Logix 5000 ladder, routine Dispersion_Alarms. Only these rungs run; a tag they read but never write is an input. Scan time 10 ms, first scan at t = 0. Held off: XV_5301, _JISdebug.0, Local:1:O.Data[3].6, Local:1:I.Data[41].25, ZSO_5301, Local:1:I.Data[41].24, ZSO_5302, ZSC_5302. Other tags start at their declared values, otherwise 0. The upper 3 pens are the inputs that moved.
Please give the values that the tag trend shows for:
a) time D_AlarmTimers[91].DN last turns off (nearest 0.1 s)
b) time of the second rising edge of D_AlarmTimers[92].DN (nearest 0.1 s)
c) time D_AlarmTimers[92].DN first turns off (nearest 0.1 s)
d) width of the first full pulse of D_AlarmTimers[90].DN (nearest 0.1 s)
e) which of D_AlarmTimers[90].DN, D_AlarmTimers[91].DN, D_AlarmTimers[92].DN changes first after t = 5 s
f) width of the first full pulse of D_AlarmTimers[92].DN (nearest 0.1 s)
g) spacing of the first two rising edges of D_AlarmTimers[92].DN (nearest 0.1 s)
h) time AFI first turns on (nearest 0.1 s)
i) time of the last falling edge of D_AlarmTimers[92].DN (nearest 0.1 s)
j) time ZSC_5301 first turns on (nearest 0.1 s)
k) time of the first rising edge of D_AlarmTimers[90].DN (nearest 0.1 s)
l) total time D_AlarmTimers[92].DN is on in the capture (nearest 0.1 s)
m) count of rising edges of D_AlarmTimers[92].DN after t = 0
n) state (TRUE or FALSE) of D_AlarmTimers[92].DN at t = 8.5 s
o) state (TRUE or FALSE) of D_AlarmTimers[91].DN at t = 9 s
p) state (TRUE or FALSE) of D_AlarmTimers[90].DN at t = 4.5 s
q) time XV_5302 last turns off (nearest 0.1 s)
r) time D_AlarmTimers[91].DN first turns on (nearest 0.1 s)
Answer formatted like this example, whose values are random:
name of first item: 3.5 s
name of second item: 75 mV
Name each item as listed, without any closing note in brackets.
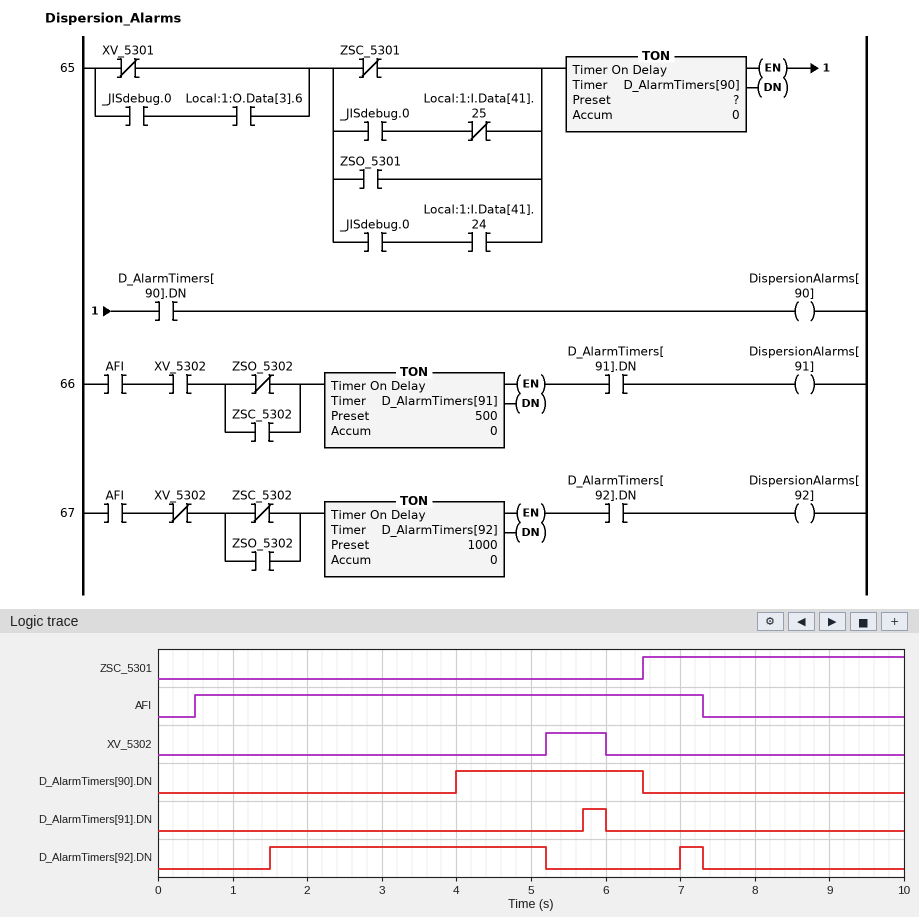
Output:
time D_AlarmTimers[91].DN last turns off: 6.0 s
time of the second rising edge of D_AlarmTimers[92].DN: 7.0 s
time D_AlarmTimers[92].DN first turns off: 5.2 s
width of the first full pulse of D_AlarmTimers[90].DN: 2.5 s
which of D_AlarmTimers[90].DN, D_AlarmTimers[91].DN, D_AlarmTimers[92].DN changes first after t = 5 s: D_AlarmTimers[92].DN
width of the first full pulse of D_AlarmTimers[92].DN: 3.7 s
spacing of the first two rising edges of D_AlarmTimers[92].DN: 5.5 s
time AFI first turns on: 0.5 s
time of the last falling edge of D_AlarmTimers[92].DN: 7.3 s
time ZSC_5301 first turns on: 6.5 s
time of the first rising edge of D_AlarmTimers[90].DN: 4.0 s
total time D_AlarmTimers[92].DN is on in the capture: 4.0 s
count of rising edges of D_AlarmTimers[92].DN after t = 0: 2
state (TRUE or FALSE) of D_AlarmTimers[92].DN at t = 8.5 s: FALSE
state (TRUE or FALSE) of D_AlarmTimers[91].DN at t = 9 s: FALSE
state (TRUE or FALSE) of D_AlarmTimers[90].DN at t = 4.5 s: TRUE
time XV_5302 last turns off: 6.0 s
time D_AlarmTimers[91].DN first turns on: 5.7 s
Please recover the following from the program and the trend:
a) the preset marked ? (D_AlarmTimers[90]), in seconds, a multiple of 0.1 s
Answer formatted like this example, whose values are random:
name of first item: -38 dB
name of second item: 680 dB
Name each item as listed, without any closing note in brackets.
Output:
the preset marked ? (D_AlarmTimers[90]), in seconds, a multiple of 0.1 s: 4.0 s
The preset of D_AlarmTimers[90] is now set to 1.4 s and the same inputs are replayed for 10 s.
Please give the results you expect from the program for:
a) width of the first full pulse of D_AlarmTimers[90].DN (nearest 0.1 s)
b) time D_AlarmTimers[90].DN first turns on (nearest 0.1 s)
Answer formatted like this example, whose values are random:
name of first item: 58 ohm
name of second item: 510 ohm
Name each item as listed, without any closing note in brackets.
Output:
width of the first full pulse of D_AlarmTimers[90].DN: 5.1 s
time D_AlarmTimers[90].DN first turns on: 1.4 s
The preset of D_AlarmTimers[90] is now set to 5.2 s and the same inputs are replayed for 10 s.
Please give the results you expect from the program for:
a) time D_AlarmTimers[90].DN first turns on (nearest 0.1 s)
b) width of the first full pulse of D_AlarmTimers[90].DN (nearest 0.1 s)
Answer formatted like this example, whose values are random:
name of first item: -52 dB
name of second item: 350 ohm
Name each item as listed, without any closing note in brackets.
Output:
time D_AlarmTimers[90].DN first turns on: 5.2 s
width of the first full pulse of D_AlarmTimers[90].DN: 1.3 s
